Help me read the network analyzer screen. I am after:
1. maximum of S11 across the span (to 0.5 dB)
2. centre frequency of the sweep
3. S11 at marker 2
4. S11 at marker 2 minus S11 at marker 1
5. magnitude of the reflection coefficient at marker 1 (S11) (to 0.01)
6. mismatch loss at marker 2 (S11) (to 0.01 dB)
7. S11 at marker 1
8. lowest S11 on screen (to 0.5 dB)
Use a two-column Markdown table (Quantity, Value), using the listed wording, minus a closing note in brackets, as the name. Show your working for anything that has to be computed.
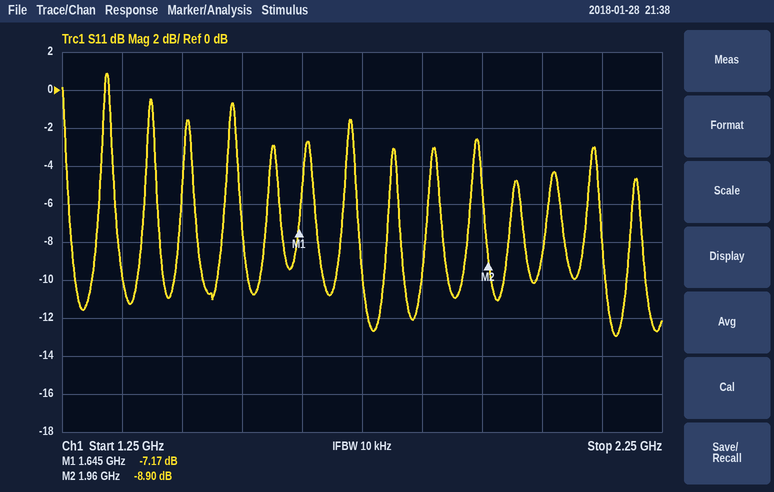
| Quantity | Value |
|---|---|
| maximum of S11 across the span | 1.0 dB |
| centre frequency of the sweep | 1.75 GHz |
| S11 at marker 2 | -8.90 dB |
| S11 at marker 2 minus S11 at marker 1 | -8.9 − (-7.17) = -1.73 dB |
| magnitude of the reflection coefficient at marker 1 (S11) | 10^(-7.17/20) ≈ 0.44 |
| mismatch loss at marker 2 (S11) | −10 log10(1 − 10^(-8.9/10)) ≈ 0.60 dB |
| S11 at marker 1 | -7.17 dB |
| lowest S11 on screen | -13.0 dB |
